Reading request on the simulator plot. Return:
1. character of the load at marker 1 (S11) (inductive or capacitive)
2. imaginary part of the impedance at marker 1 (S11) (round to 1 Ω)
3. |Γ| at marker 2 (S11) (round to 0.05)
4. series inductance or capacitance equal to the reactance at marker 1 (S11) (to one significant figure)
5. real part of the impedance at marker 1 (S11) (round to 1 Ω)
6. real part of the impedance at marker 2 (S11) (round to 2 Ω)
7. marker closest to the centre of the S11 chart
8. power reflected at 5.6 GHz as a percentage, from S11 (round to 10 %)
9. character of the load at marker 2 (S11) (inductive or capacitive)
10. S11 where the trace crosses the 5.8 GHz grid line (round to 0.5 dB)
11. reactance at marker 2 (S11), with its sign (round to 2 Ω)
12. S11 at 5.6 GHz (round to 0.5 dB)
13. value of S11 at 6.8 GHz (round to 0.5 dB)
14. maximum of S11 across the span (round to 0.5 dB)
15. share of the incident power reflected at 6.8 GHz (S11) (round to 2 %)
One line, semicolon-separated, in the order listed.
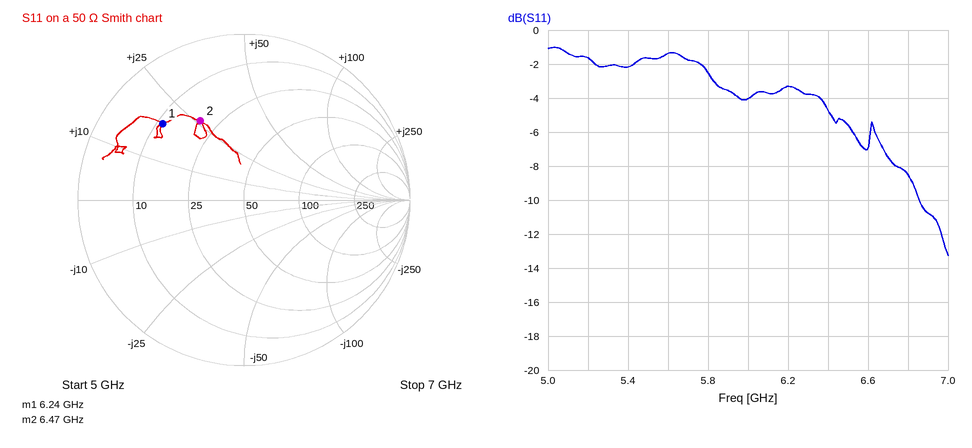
inductive; +19 Ω; 0.55; 500 pH; 11 Ω; 20 Ω; marker 2; 70 %; inductive; -2.5 dB; +26 Ω; -1.5 dB; -8.5 dB; -1.0 dB; 14 %
